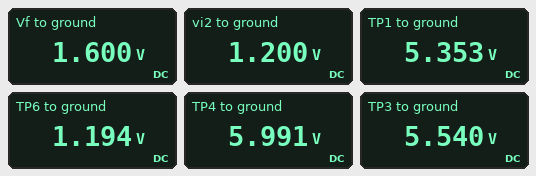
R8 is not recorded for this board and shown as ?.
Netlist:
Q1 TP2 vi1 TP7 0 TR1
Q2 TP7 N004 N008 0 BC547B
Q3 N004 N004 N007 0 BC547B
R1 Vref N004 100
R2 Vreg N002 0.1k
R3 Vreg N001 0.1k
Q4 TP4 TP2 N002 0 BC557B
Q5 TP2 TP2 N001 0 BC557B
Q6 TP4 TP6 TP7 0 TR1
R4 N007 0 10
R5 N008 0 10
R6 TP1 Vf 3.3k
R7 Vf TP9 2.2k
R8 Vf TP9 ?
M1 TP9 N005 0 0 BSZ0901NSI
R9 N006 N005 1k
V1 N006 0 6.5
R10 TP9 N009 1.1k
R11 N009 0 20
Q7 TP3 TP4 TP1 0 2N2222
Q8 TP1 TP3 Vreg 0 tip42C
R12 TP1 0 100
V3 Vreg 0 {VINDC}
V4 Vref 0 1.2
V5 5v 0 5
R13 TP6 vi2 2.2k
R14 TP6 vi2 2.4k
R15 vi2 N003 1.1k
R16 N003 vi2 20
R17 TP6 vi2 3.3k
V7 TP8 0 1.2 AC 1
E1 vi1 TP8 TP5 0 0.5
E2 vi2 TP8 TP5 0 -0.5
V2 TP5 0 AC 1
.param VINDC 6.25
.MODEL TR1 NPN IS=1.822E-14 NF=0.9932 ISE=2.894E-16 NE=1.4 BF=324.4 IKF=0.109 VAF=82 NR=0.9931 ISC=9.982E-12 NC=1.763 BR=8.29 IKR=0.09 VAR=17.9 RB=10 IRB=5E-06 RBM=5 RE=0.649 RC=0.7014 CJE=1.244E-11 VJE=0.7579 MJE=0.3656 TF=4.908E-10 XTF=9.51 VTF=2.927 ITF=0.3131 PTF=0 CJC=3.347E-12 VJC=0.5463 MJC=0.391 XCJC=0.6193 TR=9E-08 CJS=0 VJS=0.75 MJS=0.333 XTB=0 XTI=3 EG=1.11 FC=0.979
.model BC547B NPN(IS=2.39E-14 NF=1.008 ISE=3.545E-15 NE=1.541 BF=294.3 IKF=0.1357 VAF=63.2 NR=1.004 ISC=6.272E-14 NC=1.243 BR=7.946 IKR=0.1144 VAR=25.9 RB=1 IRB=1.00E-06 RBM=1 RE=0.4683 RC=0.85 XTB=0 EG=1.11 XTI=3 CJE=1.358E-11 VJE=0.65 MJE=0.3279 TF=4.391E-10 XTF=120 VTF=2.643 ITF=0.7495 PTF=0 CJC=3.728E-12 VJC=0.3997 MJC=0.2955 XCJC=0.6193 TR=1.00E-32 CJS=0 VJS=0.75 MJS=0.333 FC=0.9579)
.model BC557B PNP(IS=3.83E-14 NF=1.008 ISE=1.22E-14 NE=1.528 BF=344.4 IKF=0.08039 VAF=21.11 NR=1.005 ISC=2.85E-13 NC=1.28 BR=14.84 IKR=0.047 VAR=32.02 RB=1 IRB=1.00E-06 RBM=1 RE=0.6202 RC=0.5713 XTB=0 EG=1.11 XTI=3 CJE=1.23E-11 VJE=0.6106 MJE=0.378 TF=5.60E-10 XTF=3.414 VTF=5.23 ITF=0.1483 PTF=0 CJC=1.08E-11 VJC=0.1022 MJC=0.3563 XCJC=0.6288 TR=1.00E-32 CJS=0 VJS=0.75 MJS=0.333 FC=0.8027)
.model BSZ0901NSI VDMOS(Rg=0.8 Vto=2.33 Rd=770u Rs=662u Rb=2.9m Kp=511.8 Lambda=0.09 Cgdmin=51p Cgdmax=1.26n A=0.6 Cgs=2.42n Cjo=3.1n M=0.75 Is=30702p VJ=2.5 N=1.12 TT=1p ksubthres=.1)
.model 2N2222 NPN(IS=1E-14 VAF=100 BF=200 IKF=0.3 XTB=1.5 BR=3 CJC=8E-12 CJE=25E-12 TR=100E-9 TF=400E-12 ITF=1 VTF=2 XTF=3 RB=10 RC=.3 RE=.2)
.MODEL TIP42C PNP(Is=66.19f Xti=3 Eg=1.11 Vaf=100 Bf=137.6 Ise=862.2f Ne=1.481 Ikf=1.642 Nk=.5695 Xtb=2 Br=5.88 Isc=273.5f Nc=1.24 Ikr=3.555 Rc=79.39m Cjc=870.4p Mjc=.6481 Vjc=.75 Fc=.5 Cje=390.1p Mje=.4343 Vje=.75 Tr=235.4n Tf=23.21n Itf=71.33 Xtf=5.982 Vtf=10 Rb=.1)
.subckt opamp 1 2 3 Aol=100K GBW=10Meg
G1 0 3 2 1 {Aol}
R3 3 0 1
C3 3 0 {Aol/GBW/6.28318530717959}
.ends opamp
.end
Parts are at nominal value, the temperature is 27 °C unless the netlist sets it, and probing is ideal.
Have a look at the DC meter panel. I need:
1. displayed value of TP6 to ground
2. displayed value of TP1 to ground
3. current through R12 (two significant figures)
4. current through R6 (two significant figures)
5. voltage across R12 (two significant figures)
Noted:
1.194 V
5.353 V
54 mA
1.1 mA
5.4 V
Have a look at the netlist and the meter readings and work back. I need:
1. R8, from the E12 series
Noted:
3.9 kΩ
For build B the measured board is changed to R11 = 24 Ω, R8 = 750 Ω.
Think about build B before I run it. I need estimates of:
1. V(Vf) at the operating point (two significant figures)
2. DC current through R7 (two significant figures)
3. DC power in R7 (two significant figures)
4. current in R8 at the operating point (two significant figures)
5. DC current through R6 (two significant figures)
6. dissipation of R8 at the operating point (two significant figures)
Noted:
780 mV
350 µA
270 µW
1.0 mA
1.4 mA
800 µW
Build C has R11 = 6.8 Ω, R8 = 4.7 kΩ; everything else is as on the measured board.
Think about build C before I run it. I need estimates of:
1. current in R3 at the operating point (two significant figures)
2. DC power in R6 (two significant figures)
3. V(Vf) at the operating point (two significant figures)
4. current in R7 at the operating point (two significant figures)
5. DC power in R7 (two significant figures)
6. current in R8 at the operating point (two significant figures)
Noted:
2.4 mA
4.1 mW
1.7 V
760 µA
1.3 mW
360 µA
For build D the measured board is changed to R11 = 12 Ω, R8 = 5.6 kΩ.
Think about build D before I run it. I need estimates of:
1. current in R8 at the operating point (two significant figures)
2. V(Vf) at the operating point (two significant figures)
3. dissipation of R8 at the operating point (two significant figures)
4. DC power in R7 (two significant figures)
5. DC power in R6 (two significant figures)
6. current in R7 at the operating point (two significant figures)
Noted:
310 µA
1.7 V
540 µW
1.4 mW
4.0 mW
790 µA
